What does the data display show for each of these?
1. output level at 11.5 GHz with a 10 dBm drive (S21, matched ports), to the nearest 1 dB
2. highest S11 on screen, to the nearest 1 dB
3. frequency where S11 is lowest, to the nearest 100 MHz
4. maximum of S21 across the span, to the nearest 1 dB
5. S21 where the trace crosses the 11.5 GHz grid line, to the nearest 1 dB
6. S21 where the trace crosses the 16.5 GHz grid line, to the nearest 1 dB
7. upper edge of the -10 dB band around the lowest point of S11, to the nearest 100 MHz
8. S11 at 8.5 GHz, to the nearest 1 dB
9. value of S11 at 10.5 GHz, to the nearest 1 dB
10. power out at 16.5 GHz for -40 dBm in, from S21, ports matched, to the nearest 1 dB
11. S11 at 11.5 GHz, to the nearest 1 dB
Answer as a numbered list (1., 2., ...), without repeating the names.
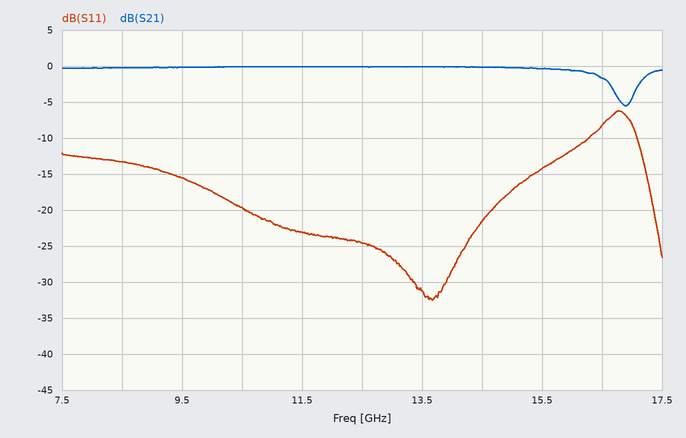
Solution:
1. 10 dBm
2. -6 dB
3. 13.7 GHz
4. 0 dB
5. 0 dB
6. -2 dB
7. 16.3 GHz
8. -13 dB
9. -20 dB
10. -42 dBm
11. -23 dB
